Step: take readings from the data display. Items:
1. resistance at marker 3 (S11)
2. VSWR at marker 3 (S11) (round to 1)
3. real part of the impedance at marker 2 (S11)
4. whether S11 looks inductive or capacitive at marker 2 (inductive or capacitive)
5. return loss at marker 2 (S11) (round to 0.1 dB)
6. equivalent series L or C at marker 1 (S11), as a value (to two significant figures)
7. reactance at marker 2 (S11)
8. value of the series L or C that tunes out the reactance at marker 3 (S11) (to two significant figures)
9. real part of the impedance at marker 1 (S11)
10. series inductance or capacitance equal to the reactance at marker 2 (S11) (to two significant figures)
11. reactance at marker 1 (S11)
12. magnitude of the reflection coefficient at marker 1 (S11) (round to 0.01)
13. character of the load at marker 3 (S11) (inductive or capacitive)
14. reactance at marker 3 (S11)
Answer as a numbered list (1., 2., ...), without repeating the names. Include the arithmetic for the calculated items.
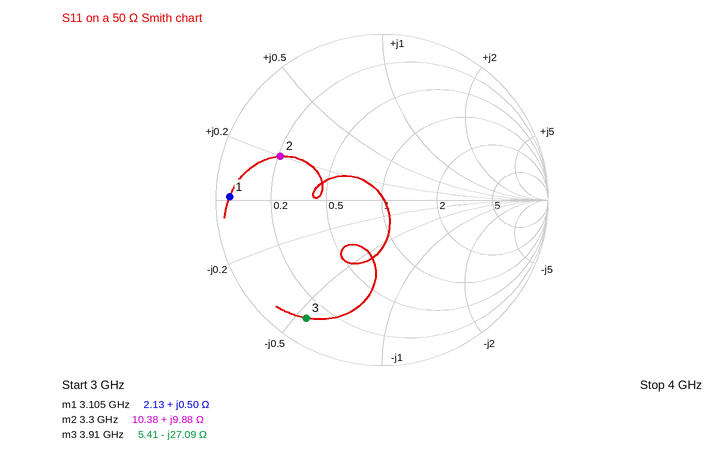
1. 5.41 Ω
2. 12
3. 10.38 Ω
4. inductive
5. 3.5 dB
6. L = 0.5 Ω/(2π × 3.105 GHz) ≈ 26 pH
7. +9.88 Ω
8. L = 27.09 Ω/(2π × 3.91 GHz) ≈ 1.1 nH
9. 2.13 Ω
10. L = 9.88 Ω/(2π × 3.3 GHz) ≈ 477 pH, so 480 pH to two significant figures
11. +0.50 Ω
12. 0.92
13. capacitive
14. -27.09 Ω
